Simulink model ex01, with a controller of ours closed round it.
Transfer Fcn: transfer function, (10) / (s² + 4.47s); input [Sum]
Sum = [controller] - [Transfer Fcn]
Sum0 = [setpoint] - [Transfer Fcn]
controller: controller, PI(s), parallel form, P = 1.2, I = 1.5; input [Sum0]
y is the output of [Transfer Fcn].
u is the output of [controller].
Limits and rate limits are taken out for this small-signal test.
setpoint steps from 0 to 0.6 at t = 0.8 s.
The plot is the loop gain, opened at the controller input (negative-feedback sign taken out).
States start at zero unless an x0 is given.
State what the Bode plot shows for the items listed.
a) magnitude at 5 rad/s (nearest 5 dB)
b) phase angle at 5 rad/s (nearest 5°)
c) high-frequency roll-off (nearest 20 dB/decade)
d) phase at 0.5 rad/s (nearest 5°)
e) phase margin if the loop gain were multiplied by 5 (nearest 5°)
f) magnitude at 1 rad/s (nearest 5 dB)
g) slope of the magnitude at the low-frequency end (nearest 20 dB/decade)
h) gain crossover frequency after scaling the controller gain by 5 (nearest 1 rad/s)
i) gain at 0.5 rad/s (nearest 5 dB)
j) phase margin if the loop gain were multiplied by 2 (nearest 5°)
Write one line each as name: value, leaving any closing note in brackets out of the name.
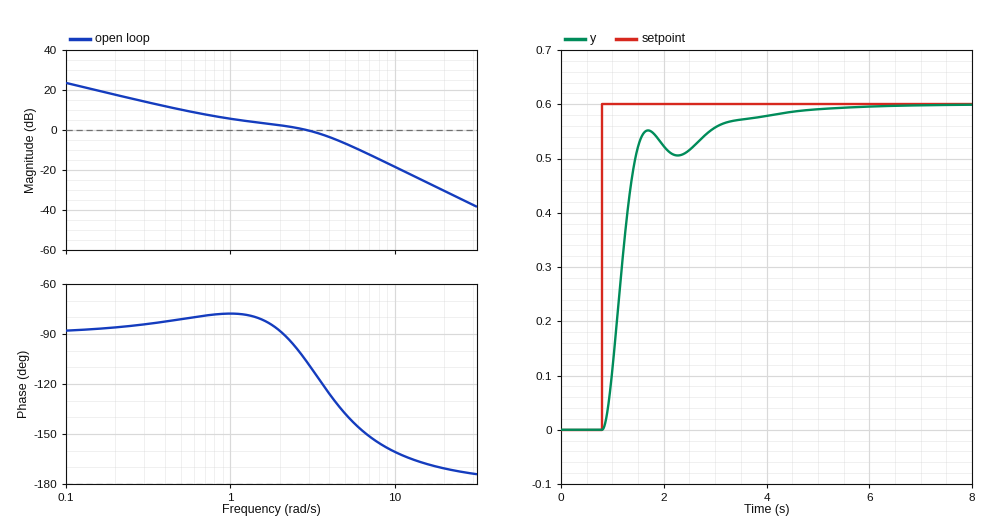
magnitude at 5 rad/s: -5 dB
phase angle at 5 rad/s: -140°
high-frequency roll-off: -40 dB/decade
phase at 0.5 rad/s: -80°
phase margin if the loop gain were multiplied by 5: 25°
magnitude at 1 rad/s: 5 dB
slope of the magnitude at the low-frequency end: -20 dB/decade
gain crossover frequency after scaling the controller gain by 5: 8 rad/s
gain at 0.5 rad/s: 10 dB
phase margin if the loop gain were multiplied by 2: 45°
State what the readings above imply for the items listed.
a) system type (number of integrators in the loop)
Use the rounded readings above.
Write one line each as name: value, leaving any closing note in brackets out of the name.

system type: 1
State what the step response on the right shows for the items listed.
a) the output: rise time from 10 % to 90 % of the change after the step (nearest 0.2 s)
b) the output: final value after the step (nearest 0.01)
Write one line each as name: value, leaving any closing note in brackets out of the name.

the output: rise time from 10 % to 90 % of the change after the step: 0.6 s
the output: final value after the step: 0.60
